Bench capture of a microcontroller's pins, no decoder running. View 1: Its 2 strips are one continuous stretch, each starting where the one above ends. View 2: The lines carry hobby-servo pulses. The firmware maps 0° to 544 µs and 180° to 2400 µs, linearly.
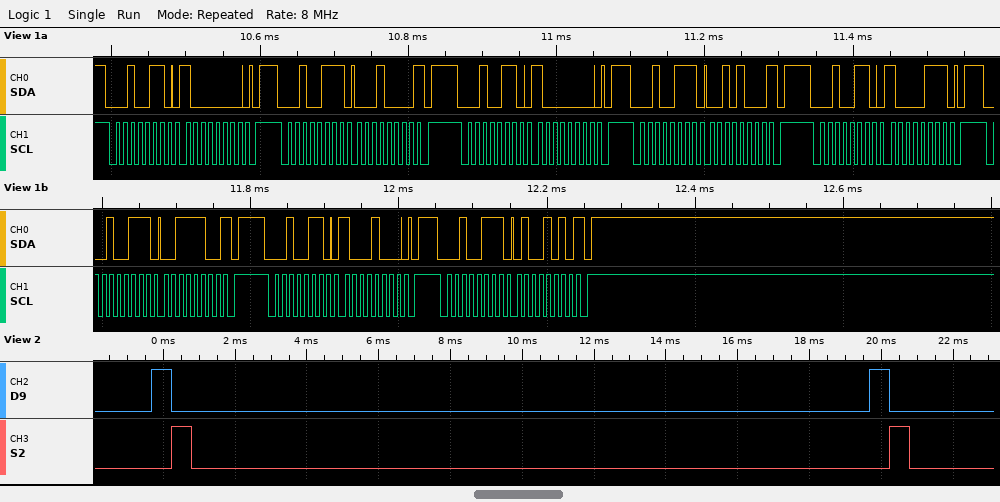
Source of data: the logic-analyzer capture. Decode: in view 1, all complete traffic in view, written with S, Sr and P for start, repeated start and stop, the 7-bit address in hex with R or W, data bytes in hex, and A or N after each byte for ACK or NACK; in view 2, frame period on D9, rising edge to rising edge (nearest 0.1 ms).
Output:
S 13W A 80 A P S 13R A 10 N P S 13W A 80 A P S 13R A 28 N P S 13W A 87 A P S 13R A 3C N P S 13W A 88 A P S 13R A 4A N P
20.0 ms
